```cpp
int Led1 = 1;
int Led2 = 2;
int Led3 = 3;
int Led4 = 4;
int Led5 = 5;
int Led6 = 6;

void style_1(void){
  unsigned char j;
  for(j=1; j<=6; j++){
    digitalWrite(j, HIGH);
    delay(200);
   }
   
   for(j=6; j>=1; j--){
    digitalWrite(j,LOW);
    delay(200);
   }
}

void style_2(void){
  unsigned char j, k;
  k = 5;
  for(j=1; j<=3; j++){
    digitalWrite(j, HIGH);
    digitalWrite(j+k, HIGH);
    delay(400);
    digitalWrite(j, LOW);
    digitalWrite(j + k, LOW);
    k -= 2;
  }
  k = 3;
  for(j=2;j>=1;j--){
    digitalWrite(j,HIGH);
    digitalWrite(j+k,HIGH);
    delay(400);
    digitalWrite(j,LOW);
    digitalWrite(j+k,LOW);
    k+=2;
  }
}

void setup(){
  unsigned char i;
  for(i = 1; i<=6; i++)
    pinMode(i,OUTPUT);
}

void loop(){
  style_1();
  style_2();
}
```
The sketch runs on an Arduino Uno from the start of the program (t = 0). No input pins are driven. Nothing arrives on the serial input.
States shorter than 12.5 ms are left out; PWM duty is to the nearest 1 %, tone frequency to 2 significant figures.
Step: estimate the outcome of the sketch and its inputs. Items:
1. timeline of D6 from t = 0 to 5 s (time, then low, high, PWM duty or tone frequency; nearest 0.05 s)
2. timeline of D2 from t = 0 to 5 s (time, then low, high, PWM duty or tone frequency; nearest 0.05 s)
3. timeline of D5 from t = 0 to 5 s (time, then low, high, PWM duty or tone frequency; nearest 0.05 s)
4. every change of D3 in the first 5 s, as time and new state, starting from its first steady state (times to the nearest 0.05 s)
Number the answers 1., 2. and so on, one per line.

1. 0 s low; 1 s high; 1.2 s low; 2.4 s high; 2.8 s low; 4 s high; 4.4 s low
2. 0 s low; 0.2 s high; 2 s low; 2.8 s high; 3.2 s low; 3.6 s high; 4 s low; 4.6 s high
3. 0 s low; 0.8 s high; 1.4 s low; 2.8 s high; 3.2 s low; 3.6 s high; 4 s low
4. 0 s low; 0.4 s high; 1.8 s low; 3.2 s high; 3.6 s low; 4.8 s high
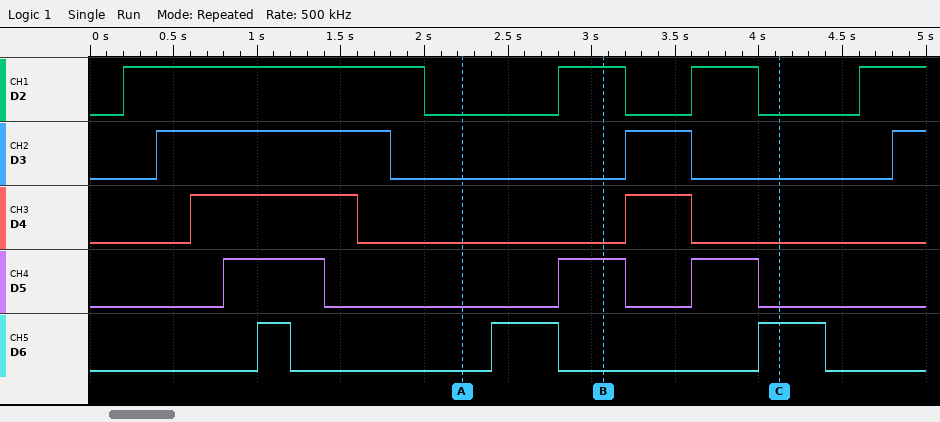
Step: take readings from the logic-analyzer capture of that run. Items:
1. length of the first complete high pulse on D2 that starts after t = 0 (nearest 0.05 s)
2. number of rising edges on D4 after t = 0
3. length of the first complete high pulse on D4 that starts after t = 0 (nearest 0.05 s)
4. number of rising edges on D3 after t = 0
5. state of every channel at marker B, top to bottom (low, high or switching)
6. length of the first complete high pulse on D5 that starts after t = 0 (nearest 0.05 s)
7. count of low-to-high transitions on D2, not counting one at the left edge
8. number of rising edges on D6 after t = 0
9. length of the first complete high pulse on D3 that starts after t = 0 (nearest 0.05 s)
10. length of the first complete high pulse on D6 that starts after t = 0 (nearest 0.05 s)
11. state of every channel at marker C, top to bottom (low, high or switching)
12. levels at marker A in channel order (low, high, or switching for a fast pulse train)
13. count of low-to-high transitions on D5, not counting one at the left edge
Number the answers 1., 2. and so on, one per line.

1. 1.80 s
2. 2
3. 1.00 s
4. 3
5. D2 high, D3 low, D4 low, D5 high, D6 low
6. 0.60 s
7. 4
8. 3
9. 1.40 s
10. 0.20 s
11. D2 low, D3 low, D4 low, D5 low, D6 high
12. D2 low, D3 low, D4 low, D5 low, D6 low
13. 3
